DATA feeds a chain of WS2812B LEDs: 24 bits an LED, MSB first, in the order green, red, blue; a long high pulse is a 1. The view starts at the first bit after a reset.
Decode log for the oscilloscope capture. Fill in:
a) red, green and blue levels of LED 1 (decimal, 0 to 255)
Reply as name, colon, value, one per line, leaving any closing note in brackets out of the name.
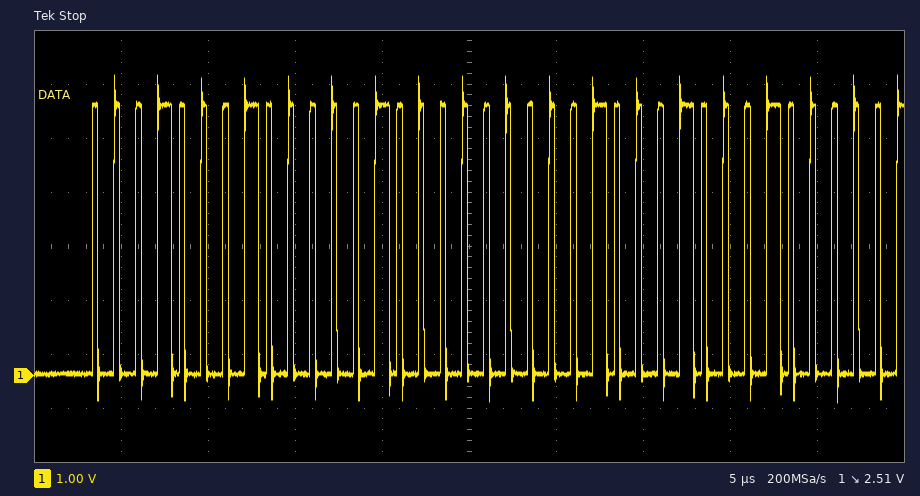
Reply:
red, green and blue levels of LED 1: 4, 17, 1
